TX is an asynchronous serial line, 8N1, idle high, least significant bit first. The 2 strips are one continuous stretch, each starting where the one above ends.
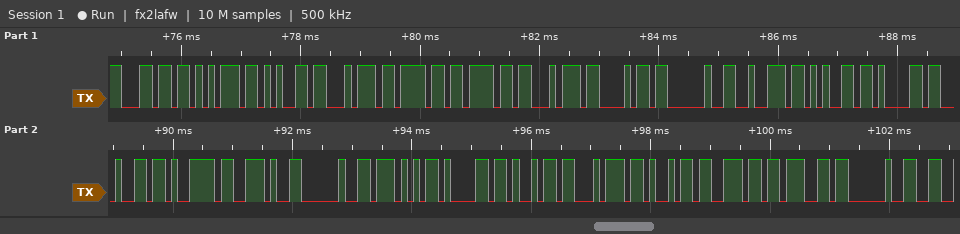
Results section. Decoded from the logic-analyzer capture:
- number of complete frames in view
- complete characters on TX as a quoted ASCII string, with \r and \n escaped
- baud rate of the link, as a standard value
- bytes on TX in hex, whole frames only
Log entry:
24
"luetooth ready. Waiting "
9600 baud
6C 75 65 74 6F 6F 74 68 20 72 65 61 64 79 2E 20 57 61 69 74 69 6E 67 20
